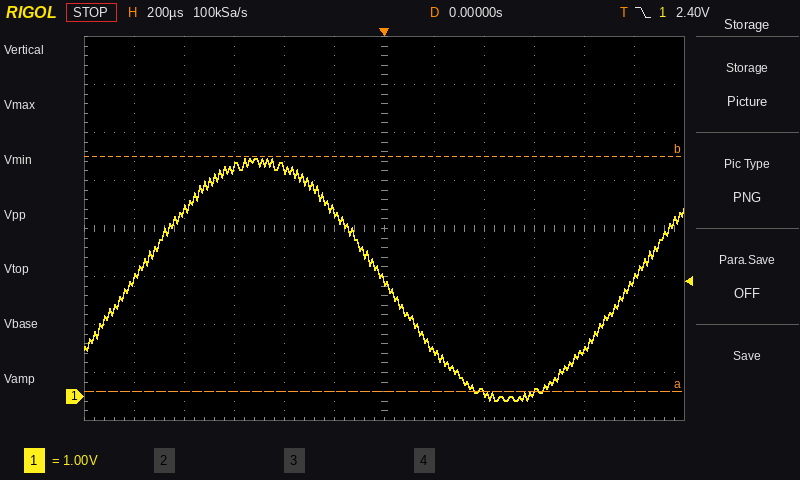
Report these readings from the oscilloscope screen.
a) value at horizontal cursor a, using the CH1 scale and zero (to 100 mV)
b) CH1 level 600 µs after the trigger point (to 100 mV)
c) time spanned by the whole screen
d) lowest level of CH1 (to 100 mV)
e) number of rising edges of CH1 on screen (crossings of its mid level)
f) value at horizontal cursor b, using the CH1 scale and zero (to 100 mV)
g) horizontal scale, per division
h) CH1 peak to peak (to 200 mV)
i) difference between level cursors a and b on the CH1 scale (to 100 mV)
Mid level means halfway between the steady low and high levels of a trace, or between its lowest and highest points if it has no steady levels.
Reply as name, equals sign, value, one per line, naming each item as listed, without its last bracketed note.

value at horizontal cursor a, using the CH1 scale and zero = 100 mV
CH1 level 600 µs after the trigger point = 100 mV
time spanned by the whole screen = 2.4 ms
lowest level of CH1 = -100 mV
number of rising edges of CH1 on screen = 2
value at horizontal cursor b, using the CH1 scale and zero = 5.0 V
horizontal scale, per division = 200 µs
CH1 peak to peak = 5.0 V
difference between level cursors a and b on the CH1 scale = 4.9 V
